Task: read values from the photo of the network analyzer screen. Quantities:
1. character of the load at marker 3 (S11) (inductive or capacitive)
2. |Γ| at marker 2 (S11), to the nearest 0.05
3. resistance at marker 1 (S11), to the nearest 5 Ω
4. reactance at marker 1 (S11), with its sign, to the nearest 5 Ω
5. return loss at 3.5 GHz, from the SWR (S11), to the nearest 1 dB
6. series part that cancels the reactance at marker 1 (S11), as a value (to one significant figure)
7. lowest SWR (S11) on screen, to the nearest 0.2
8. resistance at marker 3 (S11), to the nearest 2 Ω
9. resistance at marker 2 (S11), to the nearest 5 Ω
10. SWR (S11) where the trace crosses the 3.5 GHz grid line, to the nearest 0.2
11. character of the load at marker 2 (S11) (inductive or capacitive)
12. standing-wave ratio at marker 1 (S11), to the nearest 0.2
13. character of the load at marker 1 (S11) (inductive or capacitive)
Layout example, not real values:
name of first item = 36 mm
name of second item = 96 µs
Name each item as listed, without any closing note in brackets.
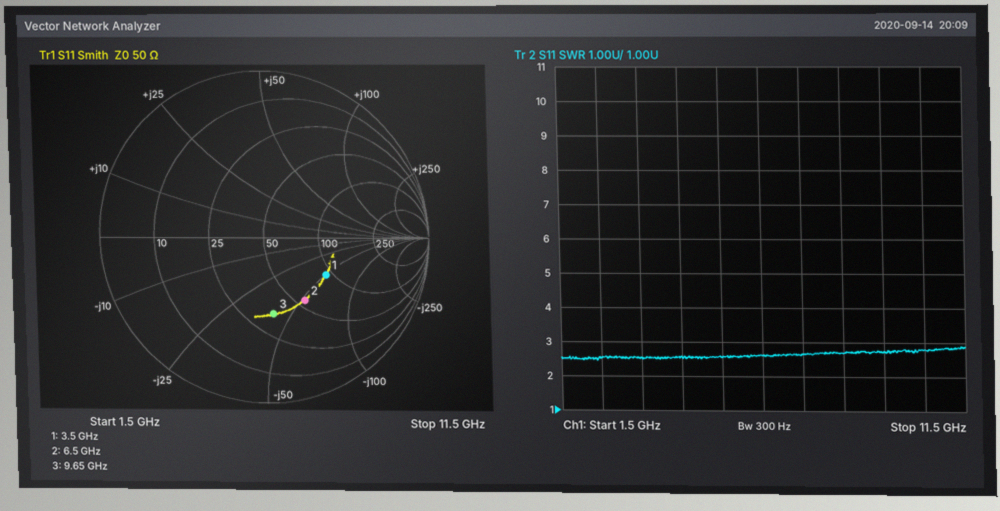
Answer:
character of the load at marker 3 (S11) = capacitive
|Γ| at marker 2 (S11), to the nearest 0.05 = 0.45
resistance at marker 1 (S11), to the nearest 5 Ω = 90 Ω
reactance at marker 1 (S11), with its sign, to the nearest 5 Ω = -50 Ω
return loss at 3.5 GHz, from the SWR (S11), to the nearest 1 dB = 7 dB
series part that cancels the reactance at marker 1 (S11), as a value = 2 nH
lowest SWR (S11) on screen, to the nearest 0.2 = 2.4
resistance at marker 3 (S11), to the nearest 2 Ω = 36 Ω
resistance at marker 2 (S11), to the nearest 5 Ω = 55 Ω
SWR (S11) where the trace crosses the 3.5 GHz grid line, to the nearest 0.2 = 2.6
character of the load at marker 2 (S11) = capacitive
standing-wave ratio at marker 1 (S11), to the nearest 0.2 = 2.6
character of the load at marker 1 (S11) = capacitive
